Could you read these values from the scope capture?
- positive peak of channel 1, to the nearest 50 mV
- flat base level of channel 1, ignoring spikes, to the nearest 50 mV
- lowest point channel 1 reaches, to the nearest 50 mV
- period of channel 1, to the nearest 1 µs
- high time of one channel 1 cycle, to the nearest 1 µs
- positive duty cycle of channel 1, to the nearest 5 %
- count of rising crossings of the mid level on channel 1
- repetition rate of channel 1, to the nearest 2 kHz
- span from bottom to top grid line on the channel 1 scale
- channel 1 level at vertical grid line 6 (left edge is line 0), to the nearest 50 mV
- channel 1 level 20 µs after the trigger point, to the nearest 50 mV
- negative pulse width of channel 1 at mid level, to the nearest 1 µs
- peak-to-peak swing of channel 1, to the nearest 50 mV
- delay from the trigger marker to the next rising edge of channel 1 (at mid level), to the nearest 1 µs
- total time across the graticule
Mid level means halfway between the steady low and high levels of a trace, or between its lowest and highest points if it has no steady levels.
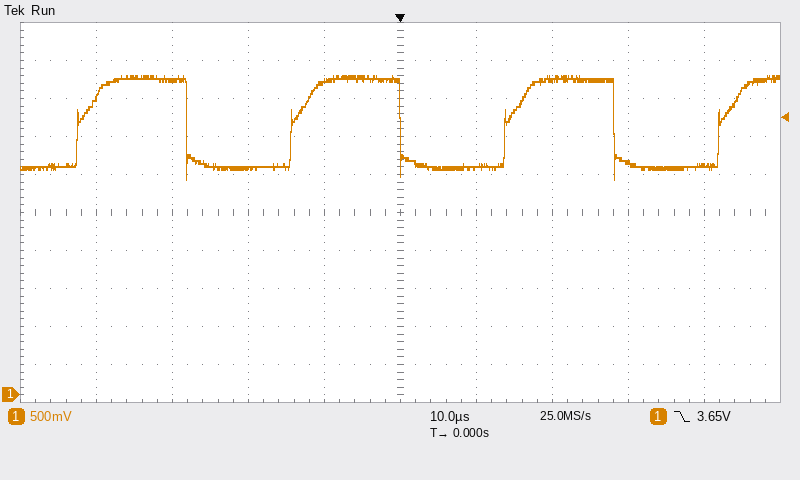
4.20 V
3.00 V
2.85 V
28 µs
14 µs
50 %
4
36 kHz
5 V
3.00 V
4.15 V
14 µs
1.35 V
14 µs
100 µs
